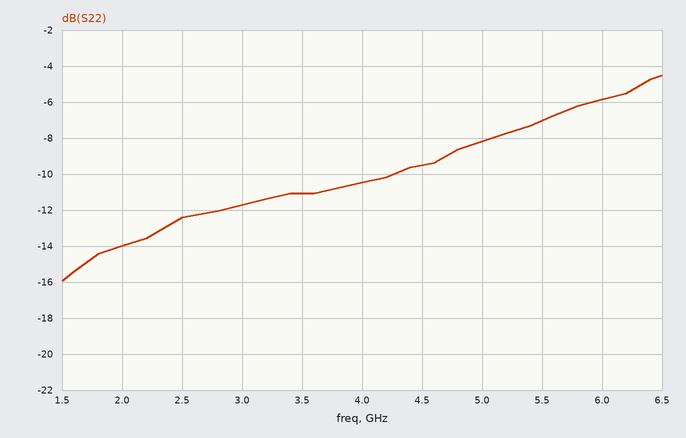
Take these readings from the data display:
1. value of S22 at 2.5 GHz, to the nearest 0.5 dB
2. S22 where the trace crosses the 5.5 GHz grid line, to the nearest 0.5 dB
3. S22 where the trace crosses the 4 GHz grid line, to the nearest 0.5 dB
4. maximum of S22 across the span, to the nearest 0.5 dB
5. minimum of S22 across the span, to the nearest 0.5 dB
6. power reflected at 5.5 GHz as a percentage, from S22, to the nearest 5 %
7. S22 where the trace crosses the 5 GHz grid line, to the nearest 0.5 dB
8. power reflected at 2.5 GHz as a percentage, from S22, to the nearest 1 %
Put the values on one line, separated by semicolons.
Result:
-12.5 dB; -7.0 dB; -10.5 dB; -4.5 dB; -16.0 dB; 20 %; -8.0 dB; 6 %
